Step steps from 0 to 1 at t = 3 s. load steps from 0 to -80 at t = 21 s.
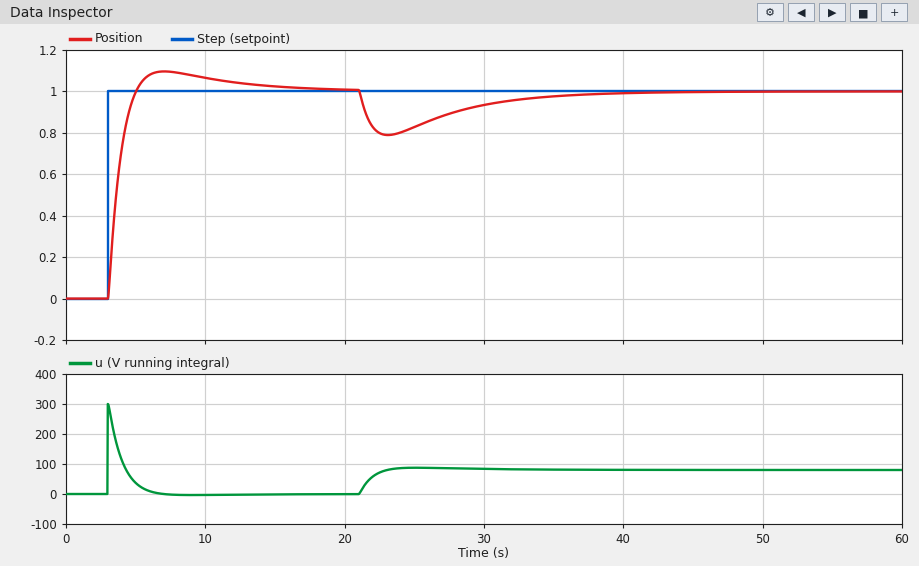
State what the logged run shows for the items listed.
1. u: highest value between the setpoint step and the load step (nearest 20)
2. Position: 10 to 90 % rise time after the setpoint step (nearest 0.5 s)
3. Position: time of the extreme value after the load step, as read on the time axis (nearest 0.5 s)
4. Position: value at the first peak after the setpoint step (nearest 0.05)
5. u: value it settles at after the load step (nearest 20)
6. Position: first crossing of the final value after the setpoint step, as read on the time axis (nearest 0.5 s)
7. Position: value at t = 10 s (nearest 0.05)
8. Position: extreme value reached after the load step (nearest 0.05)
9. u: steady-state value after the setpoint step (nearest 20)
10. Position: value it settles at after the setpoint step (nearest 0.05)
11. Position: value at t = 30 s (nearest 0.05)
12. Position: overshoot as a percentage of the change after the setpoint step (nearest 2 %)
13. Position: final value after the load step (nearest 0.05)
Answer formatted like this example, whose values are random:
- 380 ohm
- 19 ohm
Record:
- 300
- 1.5 s
- 23.0 s
- 1.10
- 80
- 5.0 s
- 1.05
- 0.80
- 0
- 1.00
- 0.95
- 10 %
- 1.00
